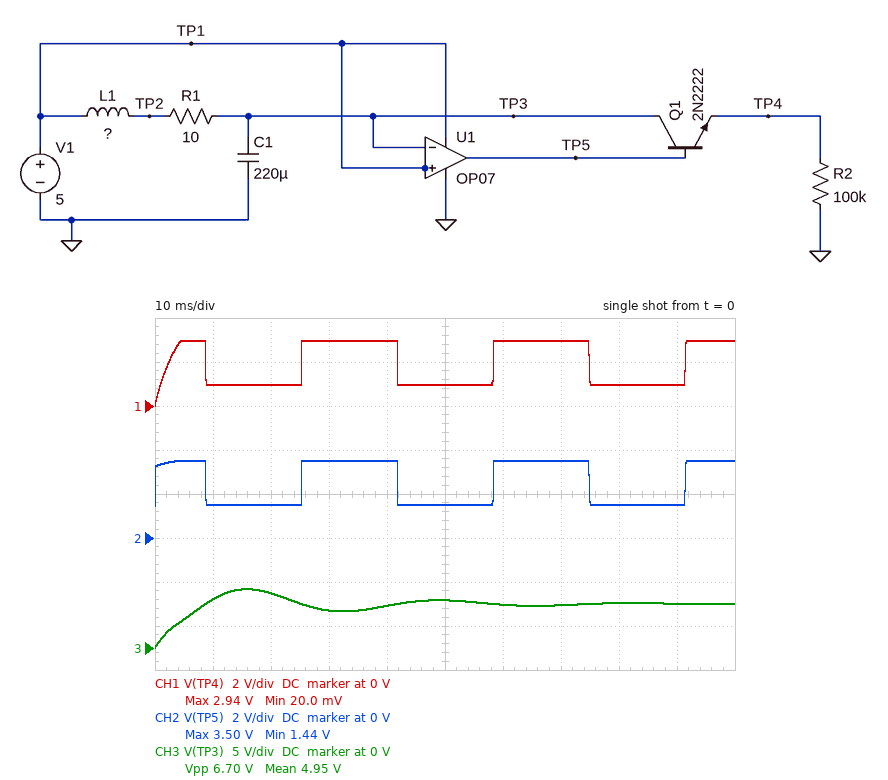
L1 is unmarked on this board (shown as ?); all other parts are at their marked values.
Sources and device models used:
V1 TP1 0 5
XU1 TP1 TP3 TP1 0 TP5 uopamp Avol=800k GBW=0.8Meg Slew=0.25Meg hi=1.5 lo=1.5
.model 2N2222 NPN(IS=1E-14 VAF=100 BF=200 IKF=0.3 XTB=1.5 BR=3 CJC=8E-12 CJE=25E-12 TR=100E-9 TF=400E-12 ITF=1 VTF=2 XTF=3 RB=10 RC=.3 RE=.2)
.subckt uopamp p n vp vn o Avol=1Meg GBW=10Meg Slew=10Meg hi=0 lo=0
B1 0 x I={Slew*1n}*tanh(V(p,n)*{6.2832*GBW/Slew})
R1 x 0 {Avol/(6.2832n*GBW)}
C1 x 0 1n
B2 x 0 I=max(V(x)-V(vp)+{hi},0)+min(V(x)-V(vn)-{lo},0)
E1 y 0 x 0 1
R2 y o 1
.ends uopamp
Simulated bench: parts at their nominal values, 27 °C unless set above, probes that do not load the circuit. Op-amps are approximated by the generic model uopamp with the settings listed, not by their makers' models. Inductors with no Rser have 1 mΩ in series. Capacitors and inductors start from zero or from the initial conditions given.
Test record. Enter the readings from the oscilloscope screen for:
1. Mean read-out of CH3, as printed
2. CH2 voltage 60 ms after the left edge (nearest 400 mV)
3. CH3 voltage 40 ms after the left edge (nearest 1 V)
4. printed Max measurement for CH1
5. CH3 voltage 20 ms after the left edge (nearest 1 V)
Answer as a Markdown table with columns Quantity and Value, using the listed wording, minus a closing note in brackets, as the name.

| Quantity | Value |
|---|---|
| Mean read-out of CH3, as printed | 4.95 V |
| CH2 voltage 60 ms after the left edge | 3.6 V |
| CH3 voltage 40 ms after the left edge | 5 V |
| printed Max measurement for CH1 | 2.94 V |
| CH3 voltage 20 ms after the left edge | 6 V |
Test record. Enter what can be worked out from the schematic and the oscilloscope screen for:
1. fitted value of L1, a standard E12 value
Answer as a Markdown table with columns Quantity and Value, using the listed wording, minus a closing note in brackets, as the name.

| Quantity | Value |
|---|---|
| fitted value of L1, a standard E12 value | 120 mH |
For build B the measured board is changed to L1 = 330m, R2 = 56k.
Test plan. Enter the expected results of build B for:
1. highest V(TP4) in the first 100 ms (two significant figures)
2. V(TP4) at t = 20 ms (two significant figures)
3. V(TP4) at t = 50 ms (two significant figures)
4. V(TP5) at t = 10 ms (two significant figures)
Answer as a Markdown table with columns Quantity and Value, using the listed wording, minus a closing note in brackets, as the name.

| Quantity | Value |
|---|---|
| highest V(TP4) in the first 100 ms | 2.9 V |
| V(TP4) at t = 20 ms | 950 mV |
| V(TP4) at t = 50 ms | 2.9 V |
| V(TP5) at t = 10 ms | 3.5 V |
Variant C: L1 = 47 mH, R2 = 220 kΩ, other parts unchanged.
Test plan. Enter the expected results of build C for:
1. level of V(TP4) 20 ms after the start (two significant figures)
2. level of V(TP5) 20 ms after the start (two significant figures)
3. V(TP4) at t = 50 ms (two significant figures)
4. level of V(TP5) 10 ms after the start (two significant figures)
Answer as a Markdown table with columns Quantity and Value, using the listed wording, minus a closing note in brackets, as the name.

| Quantity | Value |
|---|---|
| level of V(TP4) 20 ms after the start | 3.0 V |
| level of V(TP5) 20 ms after the start | 3.5 V |
| V(TP4) at t = 50 ms | 990 mV |
| level of V(TP5) 10 ms after the start | 1.5 V |
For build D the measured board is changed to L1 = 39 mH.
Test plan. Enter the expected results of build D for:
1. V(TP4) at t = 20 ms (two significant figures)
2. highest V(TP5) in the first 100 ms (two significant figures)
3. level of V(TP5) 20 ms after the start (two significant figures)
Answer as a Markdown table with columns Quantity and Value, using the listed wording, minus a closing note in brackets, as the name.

| Quantity | Value |
|---|---|
| V(TP4) at t = 20 ms | 2.9 V |
| highest V(TP5) in the first 100 ms | 3.5 V |
| level of V(TP5) 20 ms after the start | 3.5 V |
